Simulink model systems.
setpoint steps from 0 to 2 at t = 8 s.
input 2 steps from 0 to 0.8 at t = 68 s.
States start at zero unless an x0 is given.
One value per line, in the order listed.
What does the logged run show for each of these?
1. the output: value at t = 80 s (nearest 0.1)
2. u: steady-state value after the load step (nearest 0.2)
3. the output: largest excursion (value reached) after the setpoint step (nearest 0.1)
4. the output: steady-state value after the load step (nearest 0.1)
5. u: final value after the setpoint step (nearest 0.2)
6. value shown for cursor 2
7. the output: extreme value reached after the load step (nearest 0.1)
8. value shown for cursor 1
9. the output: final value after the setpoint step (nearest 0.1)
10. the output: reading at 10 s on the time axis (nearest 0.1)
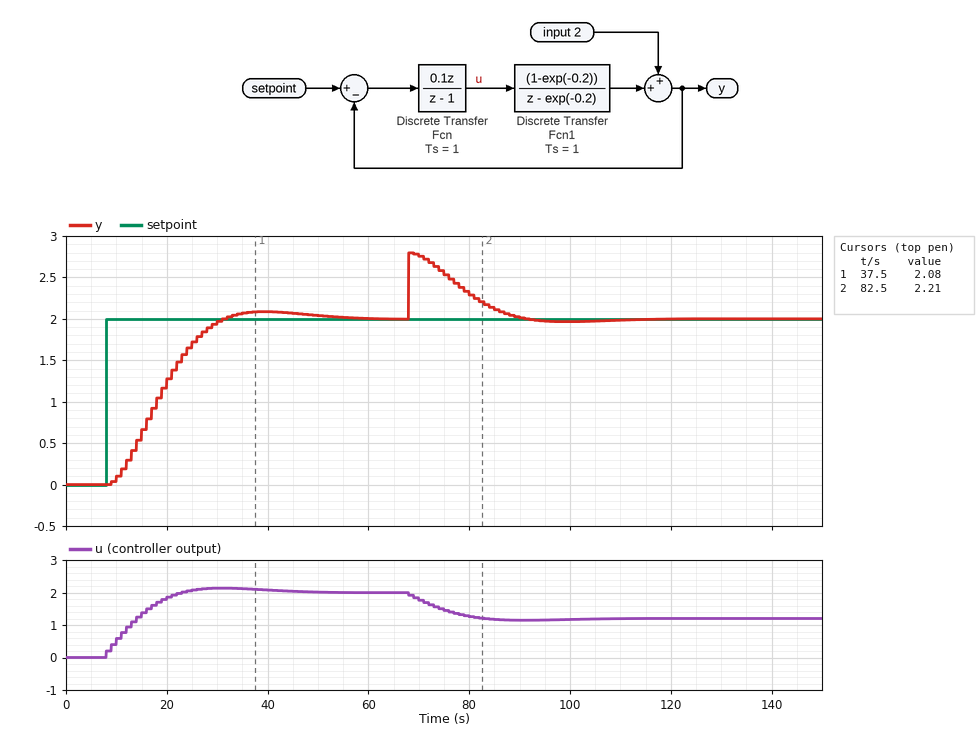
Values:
2.3
1.2
2.1
2.0
2.0
2.21
2.8
2.08
2.0
0.1
